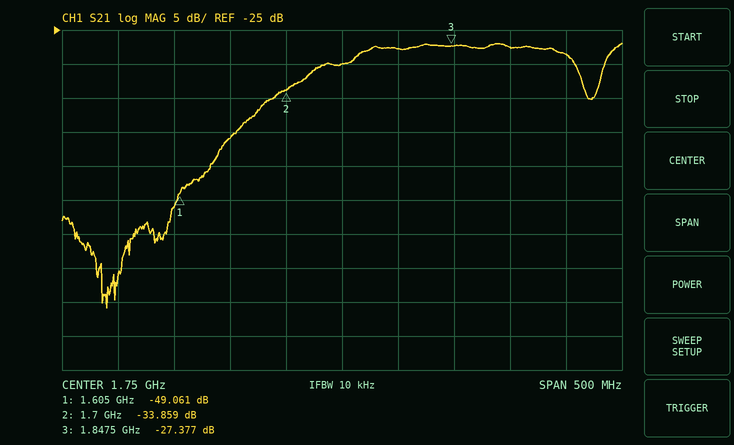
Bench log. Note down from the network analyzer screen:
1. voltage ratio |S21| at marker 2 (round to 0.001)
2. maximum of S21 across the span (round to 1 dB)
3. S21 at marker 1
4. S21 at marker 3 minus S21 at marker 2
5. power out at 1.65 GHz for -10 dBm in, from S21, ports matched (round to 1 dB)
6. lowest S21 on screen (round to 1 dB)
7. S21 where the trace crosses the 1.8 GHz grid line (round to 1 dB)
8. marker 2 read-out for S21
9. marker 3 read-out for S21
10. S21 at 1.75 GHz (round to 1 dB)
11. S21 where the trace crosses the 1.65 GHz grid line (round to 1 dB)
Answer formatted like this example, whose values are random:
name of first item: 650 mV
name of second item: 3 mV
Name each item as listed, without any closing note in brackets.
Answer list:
voltage ratio |S21| at marker 2: 0.020
maximum of S21 across the span: -27 dB
S21 at marker 1: -49.061 dB
S21 at marker 3 minus S21 at marker 2: 6.482 dB
power out at 1.65 GHz for -10 dBm in, from S21, ports matched: -51 dBm
lowest S21 on screen: -66 dB
S21 where the trace crosses the 1.8 GHz grid line: -28 dB
marker 2 read-out for S21: -33.859 dB
marker 3 read-out for S21: -27.377 dB
S21 at 1.75 GHz: -30 dB
S21 where the trace crosses the 1.65 GHz grid line: -41 dB
